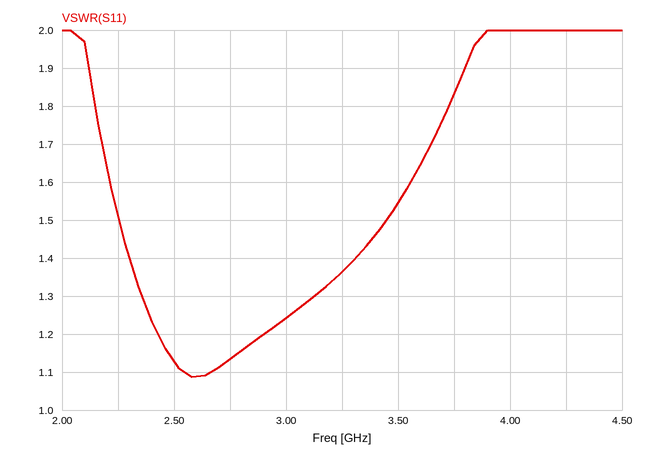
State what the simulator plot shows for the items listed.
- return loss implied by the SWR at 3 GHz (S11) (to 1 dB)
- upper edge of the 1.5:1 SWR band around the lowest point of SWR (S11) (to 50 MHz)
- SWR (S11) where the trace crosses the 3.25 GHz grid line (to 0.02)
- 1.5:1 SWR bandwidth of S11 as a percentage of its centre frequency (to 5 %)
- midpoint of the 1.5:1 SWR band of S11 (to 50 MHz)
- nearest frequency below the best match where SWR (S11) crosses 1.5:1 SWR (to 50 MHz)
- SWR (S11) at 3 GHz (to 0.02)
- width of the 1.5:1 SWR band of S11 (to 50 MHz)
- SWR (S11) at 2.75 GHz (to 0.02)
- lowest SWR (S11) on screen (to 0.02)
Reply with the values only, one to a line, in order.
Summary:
19 dB
3.45 GHz
1.36
40 %
2.85 GHz
2.25 GHz
1.24
1.20 GHz
1.14
1.08
